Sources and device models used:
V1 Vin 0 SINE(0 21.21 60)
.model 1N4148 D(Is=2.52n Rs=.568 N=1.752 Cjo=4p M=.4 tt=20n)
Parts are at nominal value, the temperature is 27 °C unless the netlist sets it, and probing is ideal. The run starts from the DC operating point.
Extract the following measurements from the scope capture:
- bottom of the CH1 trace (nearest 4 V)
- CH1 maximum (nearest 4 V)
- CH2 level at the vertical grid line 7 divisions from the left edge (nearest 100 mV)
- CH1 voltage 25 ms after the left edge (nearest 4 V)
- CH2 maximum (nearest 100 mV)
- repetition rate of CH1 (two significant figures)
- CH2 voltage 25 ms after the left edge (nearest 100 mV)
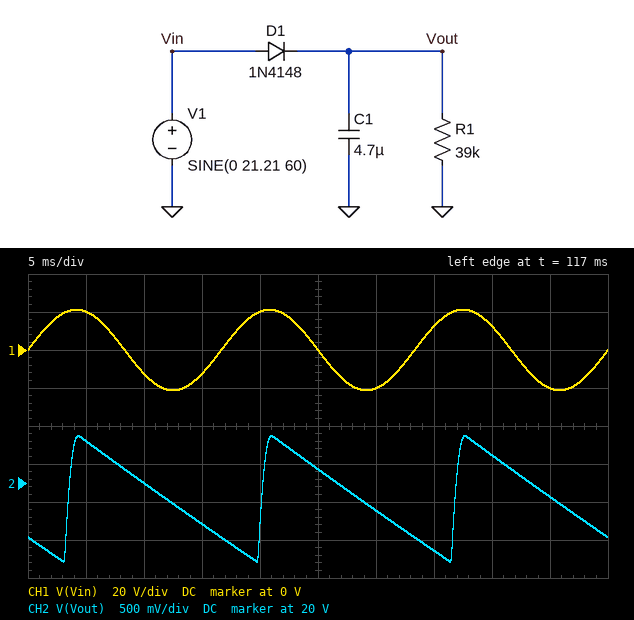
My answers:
-20 V
20 V
19.1 V
0 V
20.6 V
60 Hz
20.2 V
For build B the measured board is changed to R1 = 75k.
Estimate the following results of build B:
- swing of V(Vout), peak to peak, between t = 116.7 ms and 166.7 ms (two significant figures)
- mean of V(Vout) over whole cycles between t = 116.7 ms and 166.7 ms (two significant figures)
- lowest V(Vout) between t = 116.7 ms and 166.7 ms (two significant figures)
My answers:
890 mV
20 V
20 V
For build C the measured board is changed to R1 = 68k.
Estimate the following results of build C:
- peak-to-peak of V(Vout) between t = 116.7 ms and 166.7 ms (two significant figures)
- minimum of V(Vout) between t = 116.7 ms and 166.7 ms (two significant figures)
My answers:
980 mV
20 V
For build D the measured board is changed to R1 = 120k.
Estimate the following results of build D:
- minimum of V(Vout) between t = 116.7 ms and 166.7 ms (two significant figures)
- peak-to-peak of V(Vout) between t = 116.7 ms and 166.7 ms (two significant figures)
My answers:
20 V
570 mV
